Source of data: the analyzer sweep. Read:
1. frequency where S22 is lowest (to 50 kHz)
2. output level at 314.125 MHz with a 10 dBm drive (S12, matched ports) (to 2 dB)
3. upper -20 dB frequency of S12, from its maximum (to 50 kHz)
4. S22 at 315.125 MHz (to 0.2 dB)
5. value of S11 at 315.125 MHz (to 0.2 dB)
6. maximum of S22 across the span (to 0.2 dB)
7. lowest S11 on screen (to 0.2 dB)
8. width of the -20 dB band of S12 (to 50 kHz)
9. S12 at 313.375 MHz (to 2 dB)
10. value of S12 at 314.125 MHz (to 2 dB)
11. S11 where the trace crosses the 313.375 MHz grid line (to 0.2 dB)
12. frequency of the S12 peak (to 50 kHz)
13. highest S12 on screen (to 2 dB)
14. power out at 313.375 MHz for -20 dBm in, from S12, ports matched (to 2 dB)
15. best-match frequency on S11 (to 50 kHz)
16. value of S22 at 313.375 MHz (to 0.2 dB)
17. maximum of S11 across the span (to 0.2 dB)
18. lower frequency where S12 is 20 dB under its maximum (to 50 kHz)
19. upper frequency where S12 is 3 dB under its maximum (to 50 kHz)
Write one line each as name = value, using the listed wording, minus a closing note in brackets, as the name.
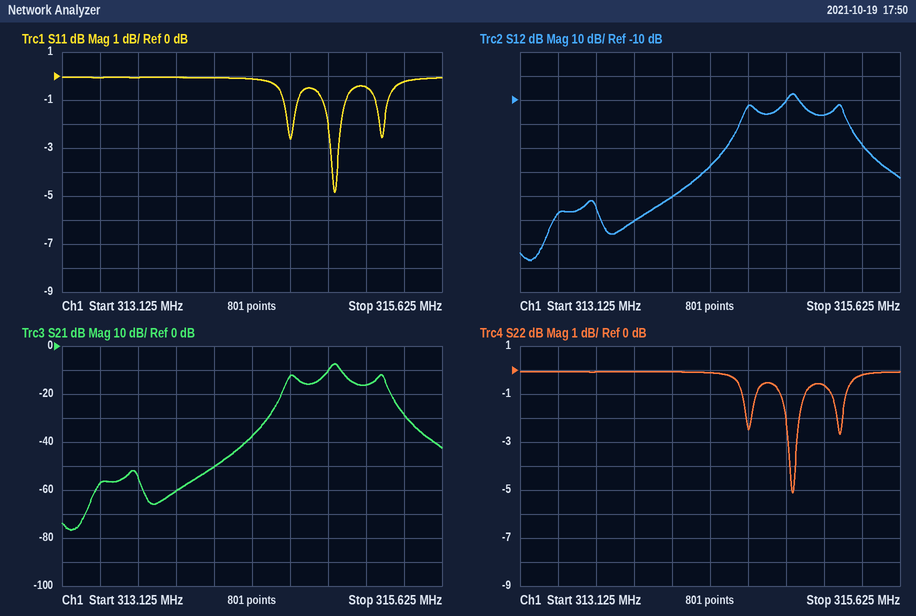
frequency where S22 is lowest = 314.90 MHz
output level at 314.125 MHz with a 10 dBm drive (S12, matched ports) = -40 dBm
upper -20 dB frequency of S12, from its maximum = 315.35 MHz
S22 at 315.125 MHz = -0.6 dB
value of S11 at 315.125 MHz = -0.4 dB
maximum of S22 across the span = 0.0 dB
lowest S11 on screen = -4.8 dB
width of the -20 dB band of S12 = 850 kHz
S12 at 313.375 MHz = -58 dB
value of S12 at 314.125 MHz = -50 dB
S11 where the trace crosses the 313.375 MHz grid line = 0.0 dB
frequency of the S12 peak = 314.90 MHz
highest S12 on screen = -8 dB
power out at 313.375 MHz for -20 dBm in, from S12, ports matched = -78 dBm
best-match frequency on S11 = 314.90 MHz
value of S22 at 313.375 MHz = 0.0 dB
maximum of S11 across the span = 0.0 dB
lower frequency where S12 is 20 dB under its maximum = 314.50 MHz
upper frequency where S12 is 3 dB under its maximum = 314.95 MHz
